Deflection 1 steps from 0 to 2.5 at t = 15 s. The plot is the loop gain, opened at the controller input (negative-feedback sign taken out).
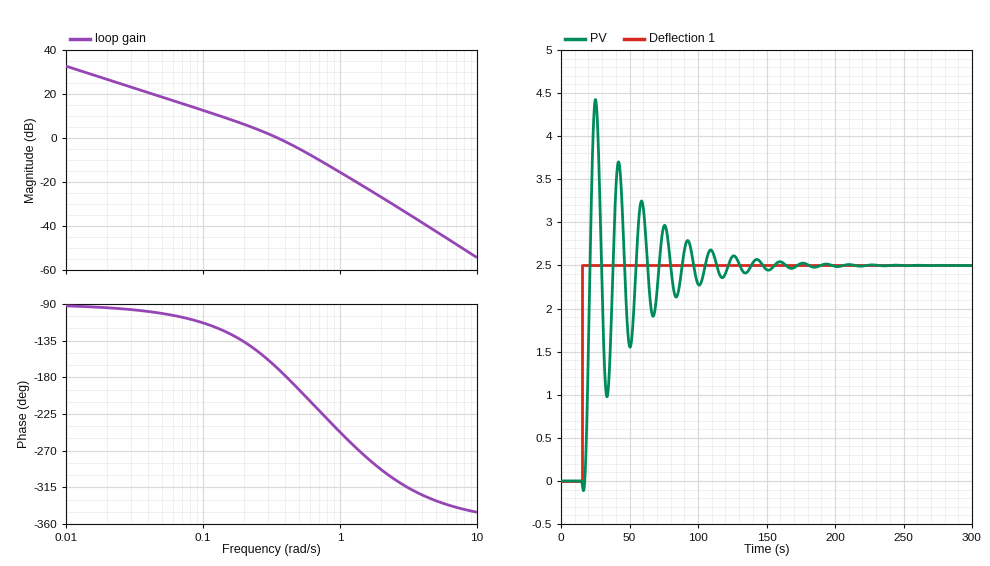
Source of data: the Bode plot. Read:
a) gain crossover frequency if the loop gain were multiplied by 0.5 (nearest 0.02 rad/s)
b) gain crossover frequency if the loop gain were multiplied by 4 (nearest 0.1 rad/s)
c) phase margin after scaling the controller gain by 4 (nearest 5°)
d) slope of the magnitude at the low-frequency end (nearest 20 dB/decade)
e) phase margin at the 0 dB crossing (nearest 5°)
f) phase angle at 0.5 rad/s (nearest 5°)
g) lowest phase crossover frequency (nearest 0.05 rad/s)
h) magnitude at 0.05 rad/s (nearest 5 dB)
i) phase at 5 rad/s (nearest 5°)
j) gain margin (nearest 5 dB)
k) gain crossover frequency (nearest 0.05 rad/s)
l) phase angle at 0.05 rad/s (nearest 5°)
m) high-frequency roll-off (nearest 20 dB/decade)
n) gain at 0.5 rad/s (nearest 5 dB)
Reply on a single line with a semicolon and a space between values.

0.20 rad/s; 0.8 rad/s; -50°; -20 dB/decade; 10°; -195°; 0.40 rad/s; 20 dB; -330°; 0 dB; 0.35 rad/s; -100°; -40 dB/decade; -5 dB
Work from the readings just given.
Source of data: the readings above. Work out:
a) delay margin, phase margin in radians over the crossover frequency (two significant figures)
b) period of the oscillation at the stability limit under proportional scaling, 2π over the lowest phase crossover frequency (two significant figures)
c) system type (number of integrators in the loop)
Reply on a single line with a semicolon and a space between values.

0.50 s; 16 s; 1
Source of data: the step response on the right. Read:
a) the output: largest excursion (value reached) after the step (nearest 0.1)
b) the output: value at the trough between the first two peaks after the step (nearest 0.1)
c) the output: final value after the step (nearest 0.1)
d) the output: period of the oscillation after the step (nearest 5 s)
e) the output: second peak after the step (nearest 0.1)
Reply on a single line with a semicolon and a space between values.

4.4; 1.0; 2.5; 15 s; 3.7
